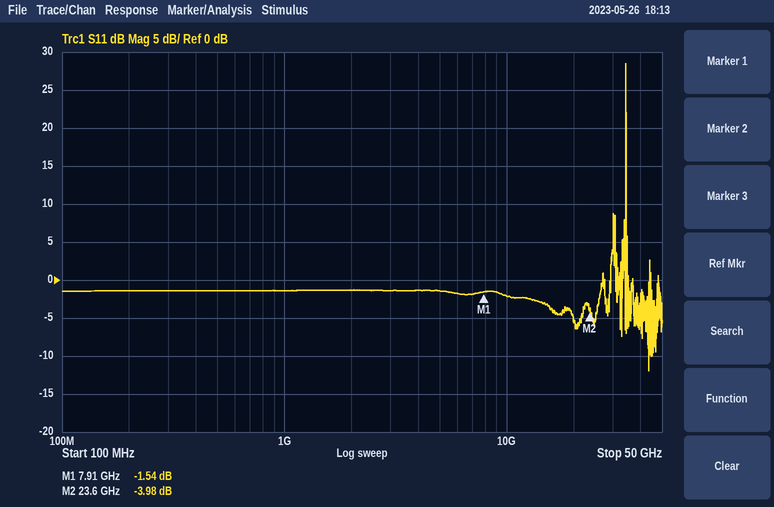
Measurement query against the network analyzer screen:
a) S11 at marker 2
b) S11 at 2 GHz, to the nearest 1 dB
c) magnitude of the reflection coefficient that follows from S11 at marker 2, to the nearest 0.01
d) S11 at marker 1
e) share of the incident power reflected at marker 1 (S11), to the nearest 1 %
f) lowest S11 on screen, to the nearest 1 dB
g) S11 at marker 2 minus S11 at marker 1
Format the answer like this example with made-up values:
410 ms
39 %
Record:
-3.98 dB
-1 dB
0.63
-1.54 dB
70 %
-12 dB
-2.44 dB
